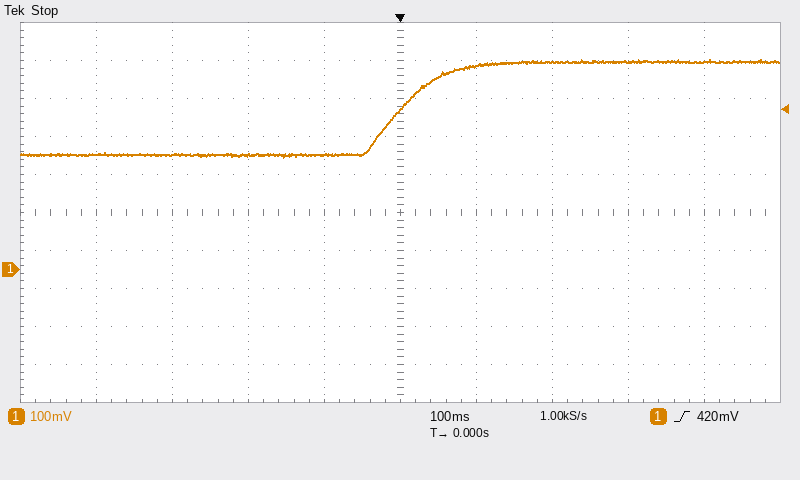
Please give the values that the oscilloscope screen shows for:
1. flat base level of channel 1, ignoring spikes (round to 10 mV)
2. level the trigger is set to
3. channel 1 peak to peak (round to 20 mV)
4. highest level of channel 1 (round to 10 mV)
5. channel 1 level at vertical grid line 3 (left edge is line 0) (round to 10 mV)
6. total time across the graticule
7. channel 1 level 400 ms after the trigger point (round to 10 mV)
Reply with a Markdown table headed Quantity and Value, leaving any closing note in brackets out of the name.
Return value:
| Quantity | Value |
|---|---|
| flat base level of channel 1, ignoring spikes | 300 mV |
| level the trigger is set to | 420 mV |
| channel 1 peak to peak | 260 mV |
| highest level of channel 1 | 550 mV |
| channel 1 level at vertical grid line 3 (left edge is line 0) | 300 mV |
| total time across the graticule | 1 s |
| channel 1 level 400 ms after the trigger point | 550 mV |
